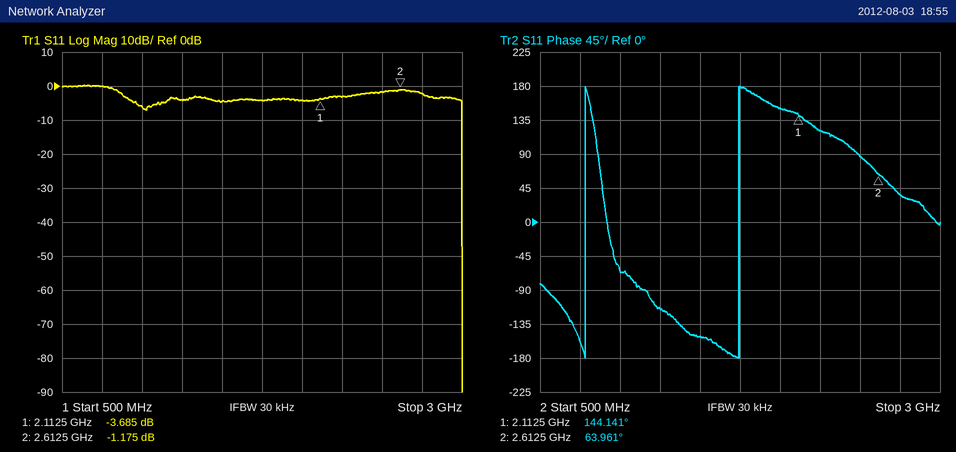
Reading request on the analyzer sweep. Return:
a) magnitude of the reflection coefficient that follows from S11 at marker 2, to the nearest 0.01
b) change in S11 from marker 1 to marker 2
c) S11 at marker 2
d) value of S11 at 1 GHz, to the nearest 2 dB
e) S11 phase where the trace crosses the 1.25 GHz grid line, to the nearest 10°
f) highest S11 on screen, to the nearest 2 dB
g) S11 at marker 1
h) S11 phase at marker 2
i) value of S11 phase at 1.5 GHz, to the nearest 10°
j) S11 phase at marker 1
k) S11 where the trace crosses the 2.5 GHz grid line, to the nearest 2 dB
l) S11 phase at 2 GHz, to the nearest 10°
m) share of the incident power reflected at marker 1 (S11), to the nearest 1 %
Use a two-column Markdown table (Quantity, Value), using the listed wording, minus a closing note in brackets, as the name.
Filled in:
| Quantity | Value |
|---|---|
| magnitude of the reflection coefficient that follows from S11 at marker 2, to the nearest 0.01 | 0.87 |
| change in S11 from marker 1 to marker 2 | 2.510 dB |
| S11 at marker 2 | -1.175 dB |
| value of S11 at 1 GHz, to the nearest 2 dB | -6 dB |
| S11 phase where the trace crosses the 1.25 GHz grid line, to the nearest 10° | -110° |
| highest S11 on screen, to the nearest 2 dB | 0 dB |
| S11 at marker 1 | -3.685 dB |
| S11 phase at marker 2 | 63.961° |
| value of S11 phase at 1.5 GHz, to the nearest 10° | -150° |
| S11 phase at marker 1 | 144.141° |
| S11 where the trace crosses the 2.5 GHz grid line, to the nearest 2 dB | -2 dB |
| S11 phase at 2 GHz, to the nearest 10° | 150° |
| share of the incident power reflected at marker 1 (S11), to the nearest 1 % | 43 % |
